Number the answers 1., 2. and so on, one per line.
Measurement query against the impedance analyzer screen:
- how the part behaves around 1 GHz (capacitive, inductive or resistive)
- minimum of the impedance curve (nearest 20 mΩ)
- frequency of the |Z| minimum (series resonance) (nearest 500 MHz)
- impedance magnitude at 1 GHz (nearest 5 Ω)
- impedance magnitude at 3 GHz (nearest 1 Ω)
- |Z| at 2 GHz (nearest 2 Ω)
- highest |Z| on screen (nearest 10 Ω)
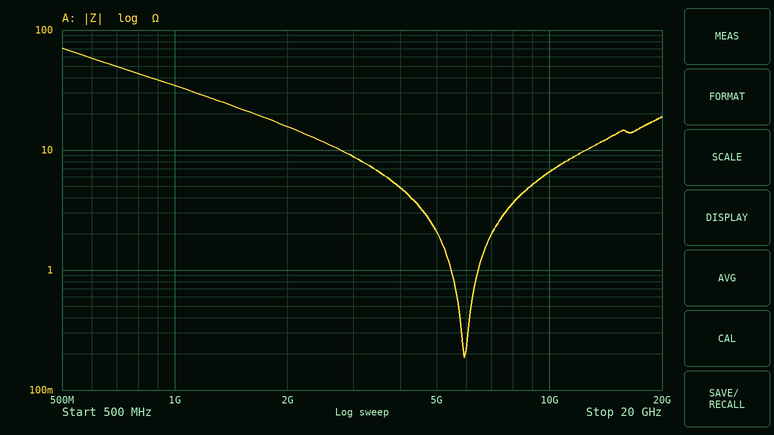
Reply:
1. capacitive
2. 180 mΩ
3. 6.0 GHz
4. 35 Ω
5. 9 Ω
6. 16 Ω
7. 70 Ω
